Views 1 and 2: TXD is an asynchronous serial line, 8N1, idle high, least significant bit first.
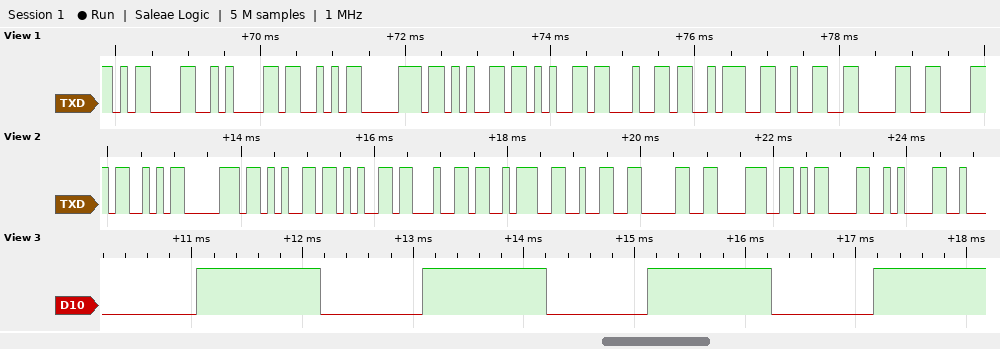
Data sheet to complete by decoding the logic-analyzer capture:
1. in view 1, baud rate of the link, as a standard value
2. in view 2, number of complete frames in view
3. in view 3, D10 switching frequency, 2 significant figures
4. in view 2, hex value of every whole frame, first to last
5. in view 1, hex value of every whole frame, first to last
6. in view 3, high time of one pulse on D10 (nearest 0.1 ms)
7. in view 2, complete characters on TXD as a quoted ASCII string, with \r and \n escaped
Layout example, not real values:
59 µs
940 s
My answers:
9600 baud
11
490 Hz
53 70 65 65 64 3A 32 30 38 0D 0A
0D 0A 53 70 65 65 64 3A 32 30
1.1 ms
"Speed:208\r\n"
